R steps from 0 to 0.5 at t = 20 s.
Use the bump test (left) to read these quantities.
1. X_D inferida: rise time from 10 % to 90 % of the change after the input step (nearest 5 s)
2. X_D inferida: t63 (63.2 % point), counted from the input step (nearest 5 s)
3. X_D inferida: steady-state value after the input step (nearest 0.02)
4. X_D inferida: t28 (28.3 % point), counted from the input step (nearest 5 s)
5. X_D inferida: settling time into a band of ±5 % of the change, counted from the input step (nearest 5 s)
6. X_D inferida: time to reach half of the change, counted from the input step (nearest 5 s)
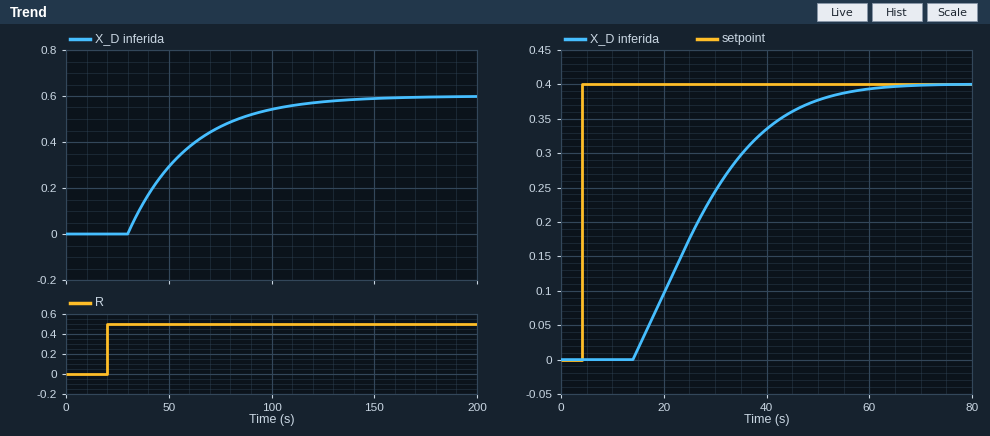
65 s
40 s
0.60
20 s
100 s
30 s
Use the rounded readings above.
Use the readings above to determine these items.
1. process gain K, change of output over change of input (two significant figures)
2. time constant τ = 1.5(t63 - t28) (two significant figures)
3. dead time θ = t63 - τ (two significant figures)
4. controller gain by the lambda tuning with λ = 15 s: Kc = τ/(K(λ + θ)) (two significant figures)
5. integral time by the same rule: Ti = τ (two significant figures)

1.2
30 s
10 s
1.0
30 s
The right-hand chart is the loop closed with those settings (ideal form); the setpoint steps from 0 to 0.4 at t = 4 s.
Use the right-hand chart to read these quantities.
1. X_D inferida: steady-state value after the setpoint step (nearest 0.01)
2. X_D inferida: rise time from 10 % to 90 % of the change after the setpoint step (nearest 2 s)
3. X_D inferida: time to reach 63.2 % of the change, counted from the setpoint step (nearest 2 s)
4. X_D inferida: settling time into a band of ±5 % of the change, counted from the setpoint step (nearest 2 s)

0.40
28 s
26 s
48 s
